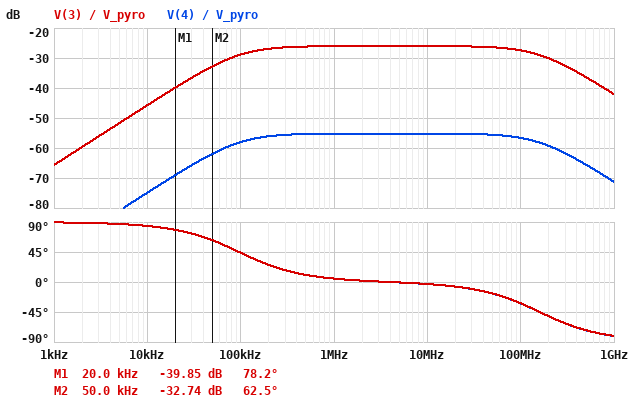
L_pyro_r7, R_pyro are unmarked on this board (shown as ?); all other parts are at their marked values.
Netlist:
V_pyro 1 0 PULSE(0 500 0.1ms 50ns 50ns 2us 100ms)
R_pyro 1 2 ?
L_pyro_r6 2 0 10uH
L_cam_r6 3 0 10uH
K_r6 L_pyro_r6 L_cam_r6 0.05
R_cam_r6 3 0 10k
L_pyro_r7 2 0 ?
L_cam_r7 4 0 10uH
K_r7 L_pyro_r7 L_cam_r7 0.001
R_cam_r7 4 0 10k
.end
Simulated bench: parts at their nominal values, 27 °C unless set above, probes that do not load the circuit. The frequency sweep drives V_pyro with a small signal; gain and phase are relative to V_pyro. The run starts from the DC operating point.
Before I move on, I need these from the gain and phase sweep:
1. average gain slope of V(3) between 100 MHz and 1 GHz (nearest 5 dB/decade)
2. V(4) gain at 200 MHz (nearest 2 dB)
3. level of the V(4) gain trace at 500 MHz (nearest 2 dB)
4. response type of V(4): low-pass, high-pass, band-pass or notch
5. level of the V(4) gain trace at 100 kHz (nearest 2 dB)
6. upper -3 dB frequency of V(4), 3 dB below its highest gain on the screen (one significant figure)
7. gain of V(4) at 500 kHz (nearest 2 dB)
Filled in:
-15 dB/decade
-60 dB
-66 dB
band-pass
-58 dB
200 MHz
-56 dB
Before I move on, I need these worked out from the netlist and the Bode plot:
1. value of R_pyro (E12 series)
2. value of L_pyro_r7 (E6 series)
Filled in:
1.5 Ω
3.3 µH
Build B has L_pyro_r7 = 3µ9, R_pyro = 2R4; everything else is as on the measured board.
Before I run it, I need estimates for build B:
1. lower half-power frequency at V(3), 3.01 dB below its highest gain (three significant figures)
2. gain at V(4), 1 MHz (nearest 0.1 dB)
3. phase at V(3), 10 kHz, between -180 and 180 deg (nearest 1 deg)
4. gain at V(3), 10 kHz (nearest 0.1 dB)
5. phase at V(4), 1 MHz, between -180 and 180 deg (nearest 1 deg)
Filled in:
136 kHz
-56.0 dB
86 deg
-48.7 dB
7 deg
